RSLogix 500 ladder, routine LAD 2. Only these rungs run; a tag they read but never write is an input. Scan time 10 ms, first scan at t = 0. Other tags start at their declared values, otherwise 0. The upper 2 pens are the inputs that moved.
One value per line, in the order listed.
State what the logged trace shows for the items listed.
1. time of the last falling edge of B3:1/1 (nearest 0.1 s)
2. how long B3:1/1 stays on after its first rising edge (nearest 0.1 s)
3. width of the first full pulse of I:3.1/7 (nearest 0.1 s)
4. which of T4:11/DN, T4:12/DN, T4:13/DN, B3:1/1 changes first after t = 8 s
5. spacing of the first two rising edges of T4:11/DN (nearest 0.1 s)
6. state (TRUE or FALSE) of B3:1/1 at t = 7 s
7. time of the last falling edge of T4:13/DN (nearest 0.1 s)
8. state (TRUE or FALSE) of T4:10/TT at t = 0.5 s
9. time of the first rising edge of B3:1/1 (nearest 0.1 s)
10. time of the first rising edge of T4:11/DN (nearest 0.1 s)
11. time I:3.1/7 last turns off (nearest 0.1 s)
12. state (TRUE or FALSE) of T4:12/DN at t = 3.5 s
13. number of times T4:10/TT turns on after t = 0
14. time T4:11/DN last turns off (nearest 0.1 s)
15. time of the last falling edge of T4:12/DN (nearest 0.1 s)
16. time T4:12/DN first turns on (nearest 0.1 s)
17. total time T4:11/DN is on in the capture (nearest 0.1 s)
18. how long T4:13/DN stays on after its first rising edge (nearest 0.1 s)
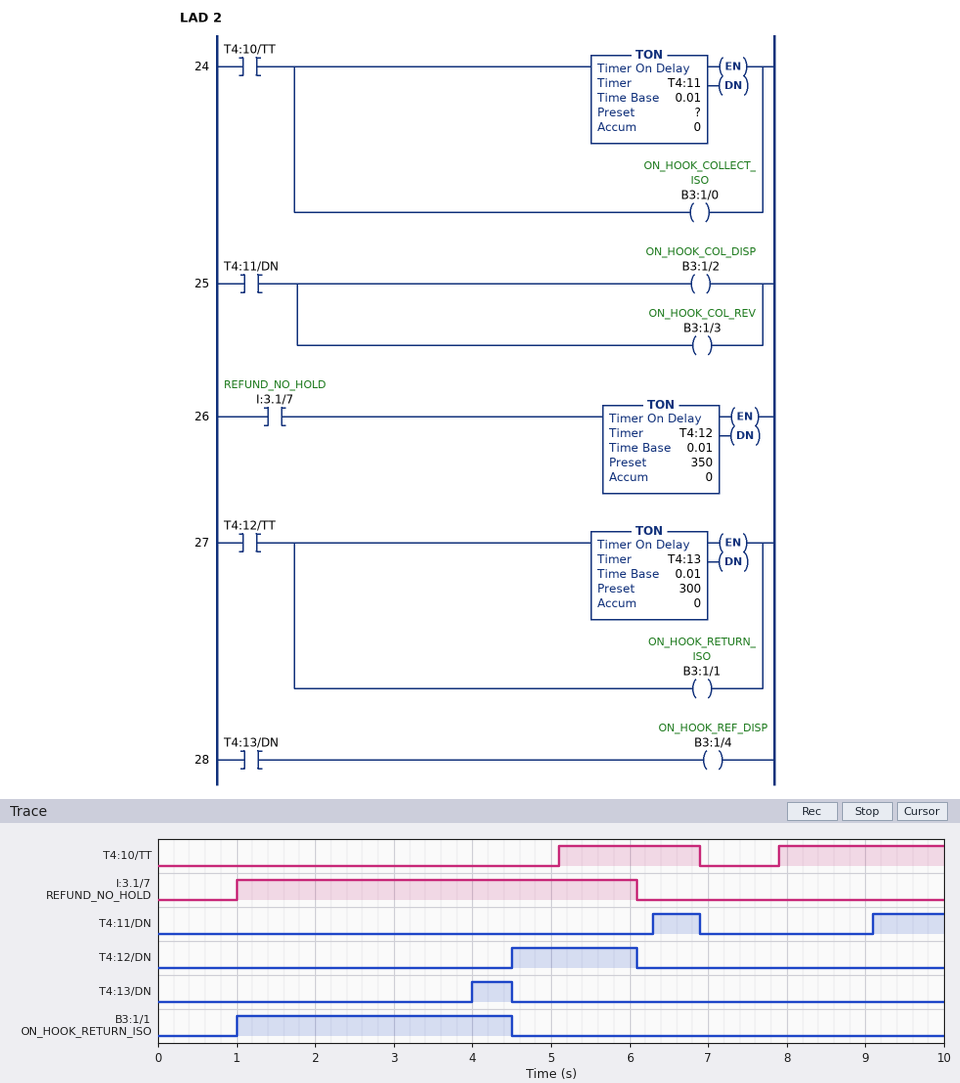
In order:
4.5 s
3.5 s
5.1 s
T4:11/DN
2.8 s
FALSE
4.5 s
FALSE
1.0 s
6.3 s
6.1 s
FALSE
2
6.9 s
6.1 s
4.5 s
1.5 s
0.5 s
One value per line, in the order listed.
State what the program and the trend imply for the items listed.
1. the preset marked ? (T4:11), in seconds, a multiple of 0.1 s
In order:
1.2 s
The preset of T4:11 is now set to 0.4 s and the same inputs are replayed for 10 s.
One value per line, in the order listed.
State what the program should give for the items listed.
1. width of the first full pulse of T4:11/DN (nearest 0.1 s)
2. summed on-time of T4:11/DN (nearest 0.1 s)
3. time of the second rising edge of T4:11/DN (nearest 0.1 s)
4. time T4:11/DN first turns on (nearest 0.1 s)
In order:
1.4 s
3.1 s
8.3 s
5.5 s
